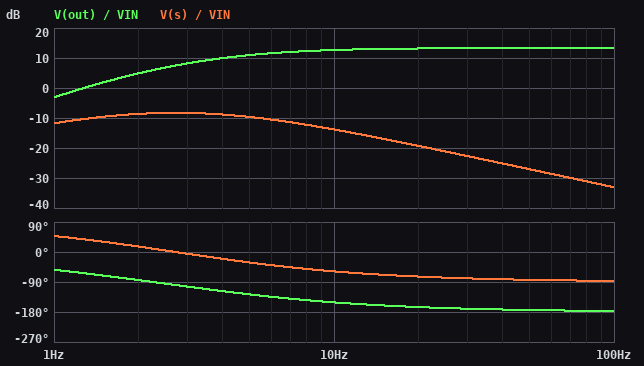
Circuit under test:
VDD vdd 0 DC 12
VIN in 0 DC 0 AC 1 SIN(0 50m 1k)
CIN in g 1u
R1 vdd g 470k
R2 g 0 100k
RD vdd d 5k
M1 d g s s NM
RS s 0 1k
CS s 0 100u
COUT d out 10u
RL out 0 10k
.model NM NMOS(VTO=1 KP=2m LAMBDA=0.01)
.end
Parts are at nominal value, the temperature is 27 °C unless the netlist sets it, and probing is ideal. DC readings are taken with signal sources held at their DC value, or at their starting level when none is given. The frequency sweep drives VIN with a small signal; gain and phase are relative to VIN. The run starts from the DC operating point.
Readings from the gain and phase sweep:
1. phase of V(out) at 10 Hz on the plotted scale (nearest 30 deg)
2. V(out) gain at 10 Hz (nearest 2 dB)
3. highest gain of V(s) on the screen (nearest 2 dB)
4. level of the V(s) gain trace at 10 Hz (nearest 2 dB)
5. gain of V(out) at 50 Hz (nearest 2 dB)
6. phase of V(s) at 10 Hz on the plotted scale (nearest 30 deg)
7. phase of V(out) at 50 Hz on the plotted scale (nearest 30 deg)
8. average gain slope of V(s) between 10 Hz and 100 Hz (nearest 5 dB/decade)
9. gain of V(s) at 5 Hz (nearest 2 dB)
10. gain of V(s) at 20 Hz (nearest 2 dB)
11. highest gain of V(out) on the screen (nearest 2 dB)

-150 deg
12 dB
-8 dB
-14 dB
14 dB
-60 deg
-180 deg
-20 dB/decade
-10 dB
-20 dB
14 dB
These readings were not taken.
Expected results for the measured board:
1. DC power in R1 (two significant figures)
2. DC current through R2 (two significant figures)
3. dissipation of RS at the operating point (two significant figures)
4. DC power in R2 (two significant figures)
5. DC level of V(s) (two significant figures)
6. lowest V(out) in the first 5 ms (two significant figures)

210 µW
21 µA
210 µW
44 µW
460 mV
-240 mV
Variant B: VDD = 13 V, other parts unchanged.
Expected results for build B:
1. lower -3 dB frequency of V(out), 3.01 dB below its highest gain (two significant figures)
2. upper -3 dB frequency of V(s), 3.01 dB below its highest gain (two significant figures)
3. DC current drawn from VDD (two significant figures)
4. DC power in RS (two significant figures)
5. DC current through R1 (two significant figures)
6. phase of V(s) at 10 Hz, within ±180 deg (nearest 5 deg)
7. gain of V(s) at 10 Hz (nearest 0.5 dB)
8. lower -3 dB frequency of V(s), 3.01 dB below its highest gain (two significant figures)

4.5 Hz
7.1 Hz
590 µA
320 µW
23 µA
-55 deg
-13.0 dB
1.1 Hz
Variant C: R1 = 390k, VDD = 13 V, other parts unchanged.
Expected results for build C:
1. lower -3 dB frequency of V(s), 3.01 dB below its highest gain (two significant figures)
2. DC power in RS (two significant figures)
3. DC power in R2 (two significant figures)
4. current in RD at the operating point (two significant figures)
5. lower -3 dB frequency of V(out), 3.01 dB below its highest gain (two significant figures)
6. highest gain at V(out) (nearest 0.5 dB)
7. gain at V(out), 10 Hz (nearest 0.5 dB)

1.2 Hz
630 µW
70 µW
800 µA
5.0 Hz
15.5 dB
14.5 dB
